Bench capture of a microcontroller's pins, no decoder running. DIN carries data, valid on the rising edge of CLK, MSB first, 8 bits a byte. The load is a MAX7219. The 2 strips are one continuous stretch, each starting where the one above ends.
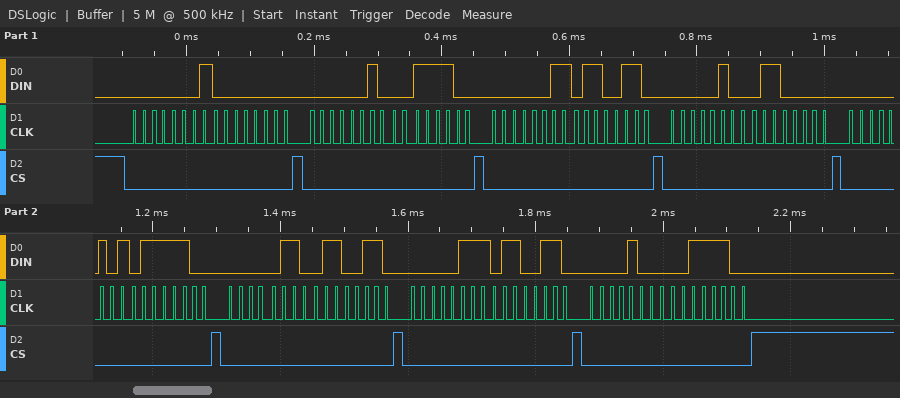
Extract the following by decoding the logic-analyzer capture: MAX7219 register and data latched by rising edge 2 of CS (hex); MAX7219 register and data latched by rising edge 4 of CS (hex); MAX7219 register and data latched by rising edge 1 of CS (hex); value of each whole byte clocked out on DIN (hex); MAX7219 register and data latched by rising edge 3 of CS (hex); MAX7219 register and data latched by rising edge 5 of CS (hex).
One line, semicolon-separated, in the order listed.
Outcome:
register 0x2, data 0x3C; register 0x4, data 0x60; register 0x1, data 0x00; 0x01 0x00 0x02 0x3C 0x03 0x66 0x04 0x60 0x05 0x7C 0x06 0x66 0x07 0x66 0x08 0x3C; register 0x3, data 0x66; register 0x5, data 0x7C
